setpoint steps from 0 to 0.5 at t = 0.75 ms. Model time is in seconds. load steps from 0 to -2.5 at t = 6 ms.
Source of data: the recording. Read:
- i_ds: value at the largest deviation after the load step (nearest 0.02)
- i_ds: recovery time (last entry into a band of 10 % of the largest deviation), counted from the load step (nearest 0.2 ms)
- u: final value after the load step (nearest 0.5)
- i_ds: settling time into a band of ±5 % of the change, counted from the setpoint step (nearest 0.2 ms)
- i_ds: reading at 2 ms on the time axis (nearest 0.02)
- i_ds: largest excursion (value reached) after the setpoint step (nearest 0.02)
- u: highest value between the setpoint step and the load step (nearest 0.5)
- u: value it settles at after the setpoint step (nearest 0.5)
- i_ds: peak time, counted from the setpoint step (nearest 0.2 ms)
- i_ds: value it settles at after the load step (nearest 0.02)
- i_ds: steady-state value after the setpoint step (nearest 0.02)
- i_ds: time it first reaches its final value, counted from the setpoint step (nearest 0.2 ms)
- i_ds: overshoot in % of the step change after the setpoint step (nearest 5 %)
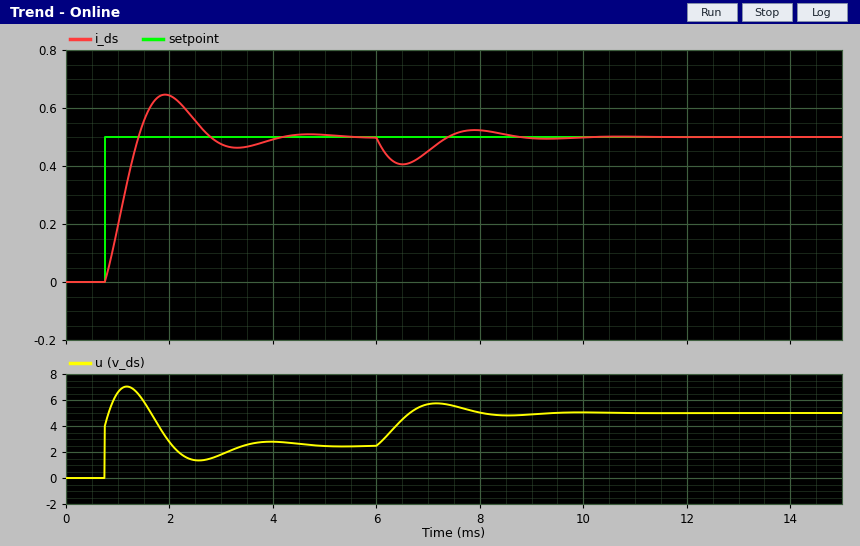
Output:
0.40
2.4 ms
5.0
3.0 ms
0.64
0.64
7.0
2.5
1.2 ms
0.50
0.50
0.6 ms
30 %
